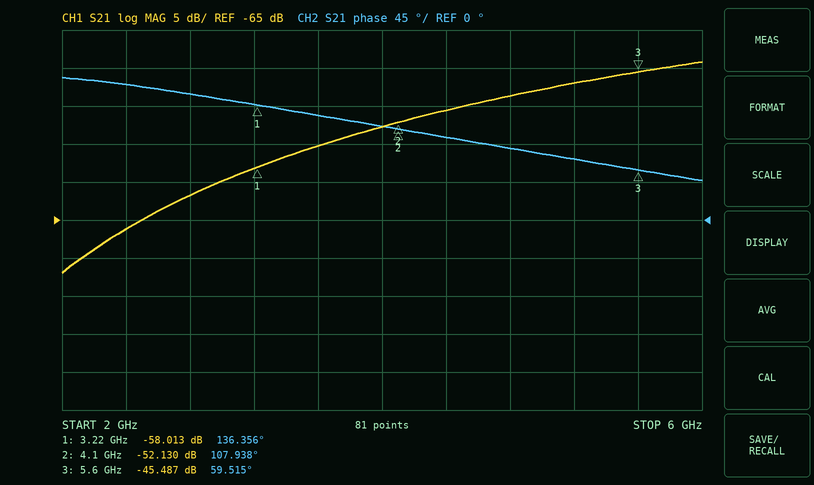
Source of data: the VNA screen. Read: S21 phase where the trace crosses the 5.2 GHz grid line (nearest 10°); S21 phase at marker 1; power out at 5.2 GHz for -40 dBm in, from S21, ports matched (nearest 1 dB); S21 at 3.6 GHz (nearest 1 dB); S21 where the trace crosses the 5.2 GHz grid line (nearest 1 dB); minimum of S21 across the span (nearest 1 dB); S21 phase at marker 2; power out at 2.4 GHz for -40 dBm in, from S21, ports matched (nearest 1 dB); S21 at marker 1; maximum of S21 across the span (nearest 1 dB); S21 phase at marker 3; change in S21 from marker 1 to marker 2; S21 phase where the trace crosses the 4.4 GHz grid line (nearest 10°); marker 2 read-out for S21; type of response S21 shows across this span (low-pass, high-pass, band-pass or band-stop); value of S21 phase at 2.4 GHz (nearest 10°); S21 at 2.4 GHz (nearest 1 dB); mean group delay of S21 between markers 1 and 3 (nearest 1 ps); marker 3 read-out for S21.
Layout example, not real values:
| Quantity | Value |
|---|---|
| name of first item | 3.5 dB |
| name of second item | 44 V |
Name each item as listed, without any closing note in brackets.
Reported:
| Quantity | Value |
|---|---|
| S21 phase where the trace crosses the 5.2 GHz grid line | 70° |
| S21 phase at marker 1 | 136.356° |
| power out at 5.2 GHz for -40 dBm in, from S21, ports matched | -87 dBm |
| S21 at 3.6 GHz | -55 dB |
| S21 where the trace crosses the 5.2 GHz grid line | -47 dB |
| minimum of S21 across the span | -72 dB |
| S21 phase at marker 2 | 107.938° |
| power out at 2.4 GHz for -40 dBm in, from S21, ports matched | -106 dBm |
| S21 at marker 1 | -58.013 dB |
| maximum of S21 across the span | -44 dB |
| S21 phase at marker 3 | 59.515° |
| change in S21 from marker 1 to marker 2 | 5.883 dB |
| S21 phase where the trace crosses the 4.4 GHz grid line | 100° |
| marker 2 read-out for S21 | -52.130 dB |
| type of response S21 shows across this span | high-pass |
| value of S21 phase at 2.4 GHz | 160° |
| S21 at 2.4 GHz | -66 dB |
| mean group delay of S21 between markers 1 and 3 | 90 ps |
| marker 3 read-out for S21 | -45.487 dB |
